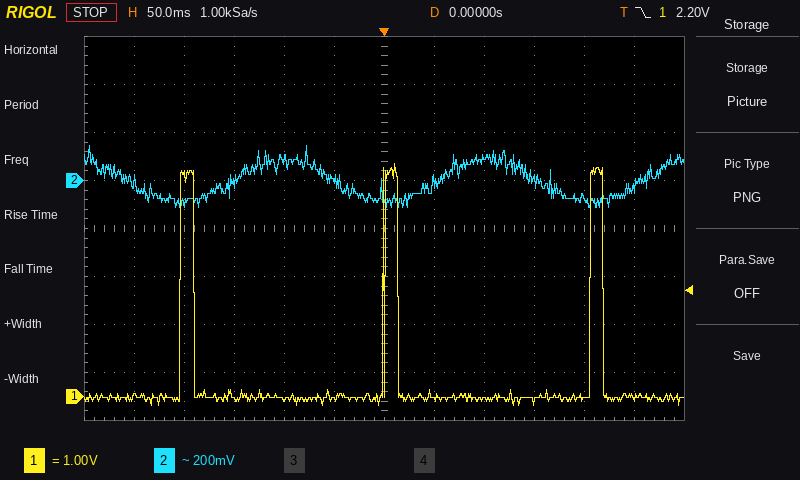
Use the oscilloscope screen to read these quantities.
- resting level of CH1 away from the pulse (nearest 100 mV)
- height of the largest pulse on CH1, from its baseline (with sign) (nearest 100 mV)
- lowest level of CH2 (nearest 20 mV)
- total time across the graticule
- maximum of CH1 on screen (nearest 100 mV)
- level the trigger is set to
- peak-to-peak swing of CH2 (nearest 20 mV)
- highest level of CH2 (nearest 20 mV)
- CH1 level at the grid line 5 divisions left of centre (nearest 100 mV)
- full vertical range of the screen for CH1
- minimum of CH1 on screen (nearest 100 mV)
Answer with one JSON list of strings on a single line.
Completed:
["0.0 V", "+4.9 V", "-120 mV", "600 ms", "4.9 V", "2.20 V", "260 mV", "140 mV", "0.0 V", "8 V", "-200 mV"]
